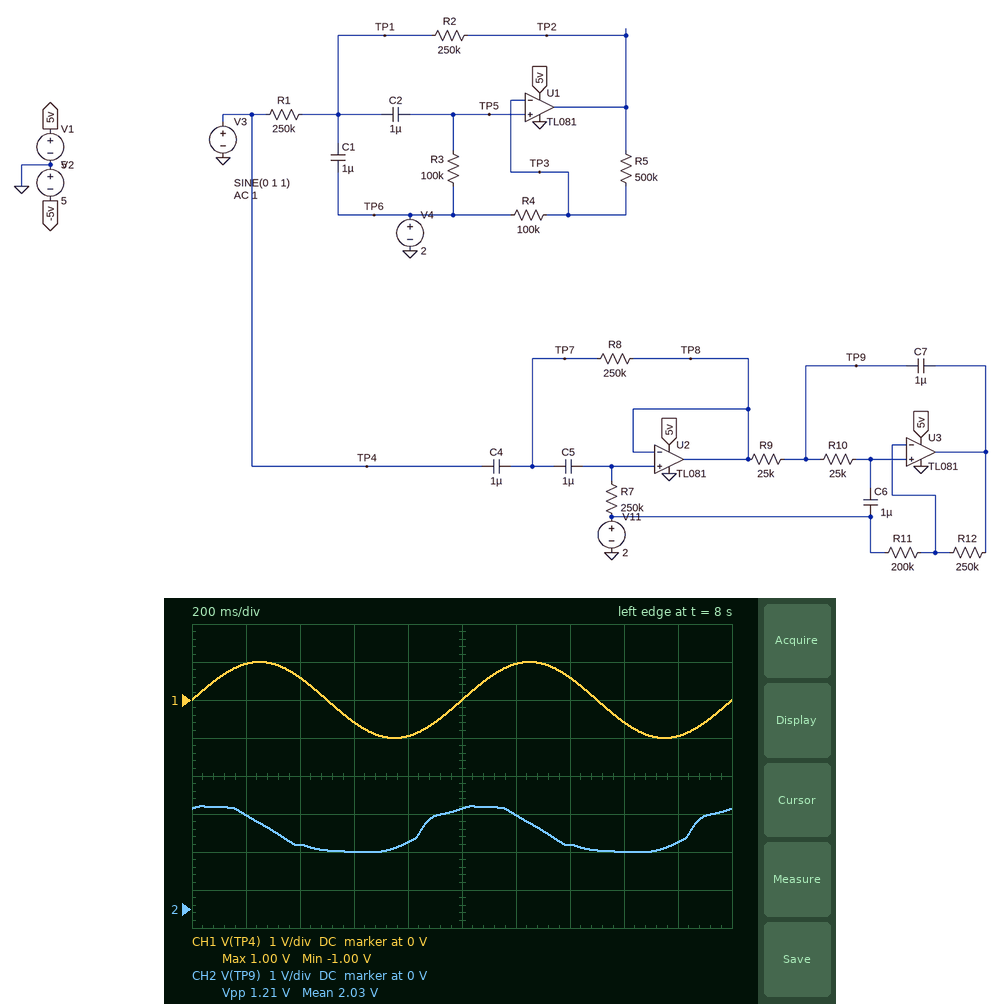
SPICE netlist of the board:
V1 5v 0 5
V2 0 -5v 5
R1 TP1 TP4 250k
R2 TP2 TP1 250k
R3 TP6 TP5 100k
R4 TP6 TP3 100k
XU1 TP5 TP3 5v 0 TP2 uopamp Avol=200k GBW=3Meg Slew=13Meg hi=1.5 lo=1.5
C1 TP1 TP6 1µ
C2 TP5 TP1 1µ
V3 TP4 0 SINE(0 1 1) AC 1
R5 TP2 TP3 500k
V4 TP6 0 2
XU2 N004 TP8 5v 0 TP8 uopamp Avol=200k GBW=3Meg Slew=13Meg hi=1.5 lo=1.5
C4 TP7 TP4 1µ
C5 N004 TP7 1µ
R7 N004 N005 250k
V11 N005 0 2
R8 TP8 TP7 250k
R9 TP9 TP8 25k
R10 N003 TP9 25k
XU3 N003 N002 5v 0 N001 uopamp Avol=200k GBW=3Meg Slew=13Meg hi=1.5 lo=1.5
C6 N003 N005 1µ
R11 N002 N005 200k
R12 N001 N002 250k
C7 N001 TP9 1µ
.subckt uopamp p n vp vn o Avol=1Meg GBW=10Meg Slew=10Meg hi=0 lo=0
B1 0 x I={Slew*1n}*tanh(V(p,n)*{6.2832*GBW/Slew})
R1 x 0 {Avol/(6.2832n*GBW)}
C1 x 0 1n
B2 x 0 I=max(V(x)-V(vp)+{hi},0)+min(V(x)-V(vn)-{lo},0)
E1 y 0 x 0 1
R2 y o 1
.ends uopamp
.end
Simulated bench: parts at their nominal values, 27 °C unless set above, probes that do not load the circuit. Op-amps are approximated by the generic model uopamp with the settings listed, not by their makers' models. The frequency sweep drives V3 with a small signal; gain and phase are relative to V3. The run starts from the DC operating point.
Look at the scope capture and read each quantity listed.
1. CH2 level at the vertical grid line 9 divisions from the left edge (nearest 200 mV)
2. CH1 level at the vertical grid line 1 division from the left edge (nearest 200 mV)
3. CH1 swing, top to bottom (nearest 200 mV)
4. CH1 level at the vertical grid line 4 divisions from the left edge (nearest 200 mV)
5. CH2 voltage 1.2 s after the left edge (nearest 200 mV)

1.8 V
1.0 V
2.0 V
-1.0 V
2.4 V
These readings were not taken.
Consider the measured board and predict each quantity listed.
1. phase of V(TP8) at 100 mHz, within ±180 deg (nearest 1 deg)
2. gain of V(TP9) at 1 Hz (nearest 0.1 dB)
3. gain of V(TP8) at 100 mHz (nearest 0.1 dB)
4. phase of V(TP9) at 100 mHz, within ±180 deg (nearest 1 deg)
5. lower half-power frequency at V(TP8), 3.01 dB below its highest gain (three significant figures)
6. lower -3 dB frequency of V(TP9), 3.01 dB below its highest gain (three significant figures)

162 deg
-2.7 dB
-32.4 dB
162 deg
989 mHz
3.43 Hz
